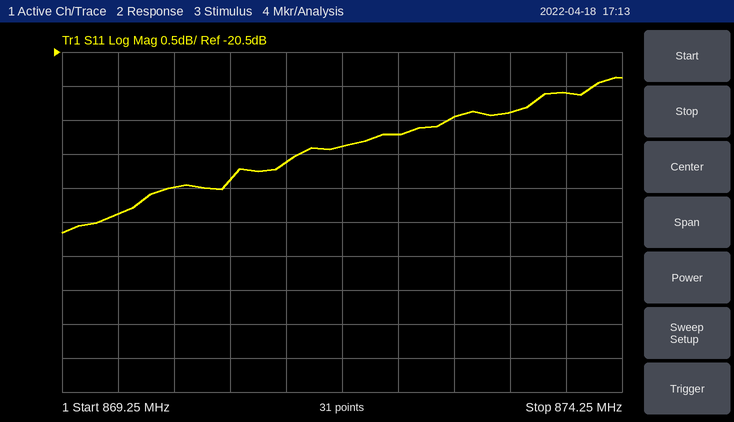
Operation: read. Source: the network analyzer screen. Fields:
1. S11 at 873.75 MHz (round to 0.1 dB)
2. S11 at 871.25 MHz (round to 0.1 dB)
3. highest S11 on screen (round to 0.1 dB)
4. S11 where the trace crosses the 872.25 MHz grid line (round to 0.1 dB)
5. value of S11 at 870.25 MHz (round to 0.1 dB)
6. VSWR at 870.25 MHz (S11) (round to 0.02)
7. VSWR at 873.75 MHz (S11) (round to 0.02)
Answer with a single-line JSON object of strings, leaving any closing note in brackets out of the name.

{"S11 at 873.75 MHz": "-21.1 dB", "S11 at 871.25 MHz": "-22.1 dB", "highest S11 on screen": "-20.9 dB", "S11 where the trace crosses the 872.25 MHz grid line": "-21.7 dB", "value of S11 at 870.25 MHz": "-22.5 dB", "VSWR at 870.25 MHz (S11)": "1.16", "VSWR at 873.75 MHz (S11)": "1.20"}
